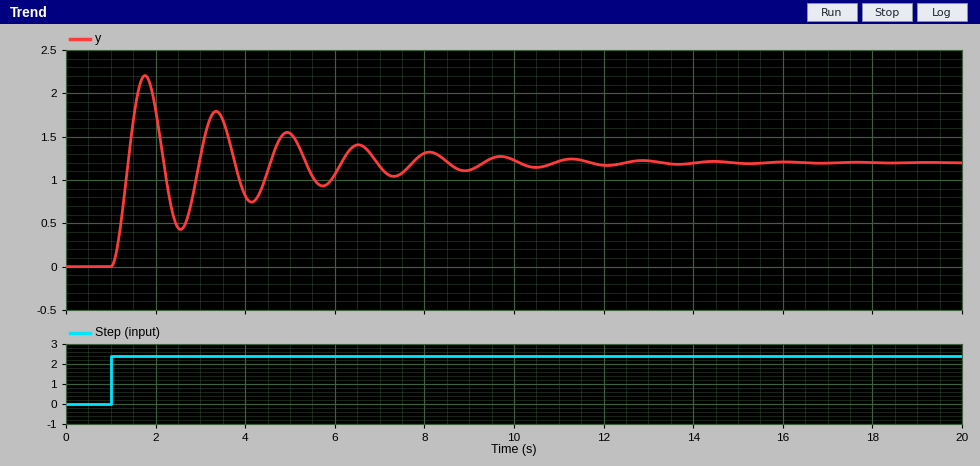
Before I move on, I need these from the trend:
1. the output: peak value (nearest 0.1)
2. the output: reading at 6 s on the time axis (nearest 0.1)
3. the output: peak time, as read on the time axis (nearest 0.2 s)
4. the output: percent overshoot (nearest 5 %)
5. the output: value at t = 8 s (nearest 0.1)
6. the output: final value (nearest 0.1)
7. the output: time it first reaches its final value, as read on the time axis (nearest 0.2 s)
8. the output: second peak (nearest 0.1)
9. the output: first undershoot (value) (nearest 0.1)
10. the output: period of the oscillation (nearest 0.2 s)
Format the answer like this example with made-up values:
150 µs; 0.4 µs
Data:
2.2; 1.1; 1.8 s; 85 %; 1.3; 1.2; 1.4 s; 1.8; 0.4; 1.6 s
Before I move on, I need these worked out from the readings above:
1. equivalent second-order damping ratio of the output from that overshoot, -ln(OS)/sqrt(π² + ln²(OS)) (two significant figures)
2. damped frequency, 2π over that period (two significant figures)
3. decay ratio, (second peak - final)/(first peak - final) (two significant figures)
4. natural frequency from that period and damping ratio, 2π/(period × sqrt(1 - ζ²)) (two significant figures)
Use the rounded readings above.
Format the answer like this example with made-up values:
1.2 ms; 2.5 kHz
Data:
0.052; 3.9 rad/s; 0.60; 3.9 rad/s
